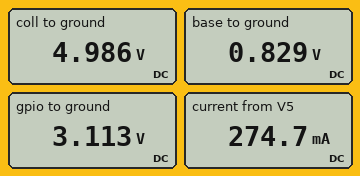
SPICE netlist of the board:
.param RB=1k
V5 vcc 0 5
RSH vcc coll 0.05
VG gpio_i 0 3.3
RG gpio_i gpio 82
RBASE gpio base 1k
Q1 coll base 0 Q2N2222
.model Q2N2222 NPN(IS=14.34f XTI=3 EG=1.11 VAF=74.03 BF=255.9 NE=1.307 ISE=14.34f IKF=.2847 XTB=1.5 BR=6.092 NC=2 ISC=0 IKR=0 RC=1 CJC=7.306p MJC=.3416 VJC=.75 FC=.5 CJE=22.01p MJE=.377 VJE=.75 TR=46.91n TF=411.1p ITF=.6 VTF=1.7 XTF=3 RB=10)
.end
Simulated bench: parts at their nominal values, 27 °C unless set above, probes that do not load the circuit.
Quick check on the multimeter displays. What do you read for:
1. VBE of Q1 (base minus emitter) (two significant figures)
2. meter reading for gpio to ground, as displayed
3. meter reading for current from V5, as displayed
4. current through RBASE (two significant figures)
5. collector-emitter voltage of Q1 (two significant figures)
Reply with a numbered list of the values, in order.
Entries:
1. 830 mV
2. 3.113 V
3. 274.7 mA
4. 2.3 mA
5. 5.0 V
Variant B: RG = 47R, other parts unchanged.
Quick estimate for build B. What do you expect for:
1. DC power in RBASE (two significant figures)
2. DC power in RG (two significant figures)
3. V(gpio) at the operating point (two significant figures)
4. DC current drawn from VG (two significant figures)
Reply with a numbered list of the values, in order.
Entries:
1. 5.6 mW
2. 260 µW
3. 3.2 V
4. 2.4 mA
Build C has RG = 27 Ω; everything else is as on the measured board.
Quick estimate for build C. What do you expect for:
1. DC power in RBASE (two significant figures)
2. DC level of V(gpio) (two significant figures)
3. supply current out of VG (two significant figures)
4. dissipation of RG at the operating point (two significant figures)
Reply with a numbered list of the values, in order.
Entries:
1. 5.8 mW
2. 3.2 V
3. 2.4 mA
4. 160 µW
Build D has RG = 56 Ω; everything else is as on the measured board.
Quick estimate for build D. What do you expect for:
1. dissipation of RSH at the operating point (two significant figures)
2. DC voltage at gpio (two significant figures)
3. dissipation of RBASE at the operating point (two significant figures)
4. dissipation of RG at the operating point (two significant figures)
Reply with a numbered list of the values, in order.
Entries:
1. 3.9 mW
2. 3.2 V
3. 5.5 mW
4. 310 µW
